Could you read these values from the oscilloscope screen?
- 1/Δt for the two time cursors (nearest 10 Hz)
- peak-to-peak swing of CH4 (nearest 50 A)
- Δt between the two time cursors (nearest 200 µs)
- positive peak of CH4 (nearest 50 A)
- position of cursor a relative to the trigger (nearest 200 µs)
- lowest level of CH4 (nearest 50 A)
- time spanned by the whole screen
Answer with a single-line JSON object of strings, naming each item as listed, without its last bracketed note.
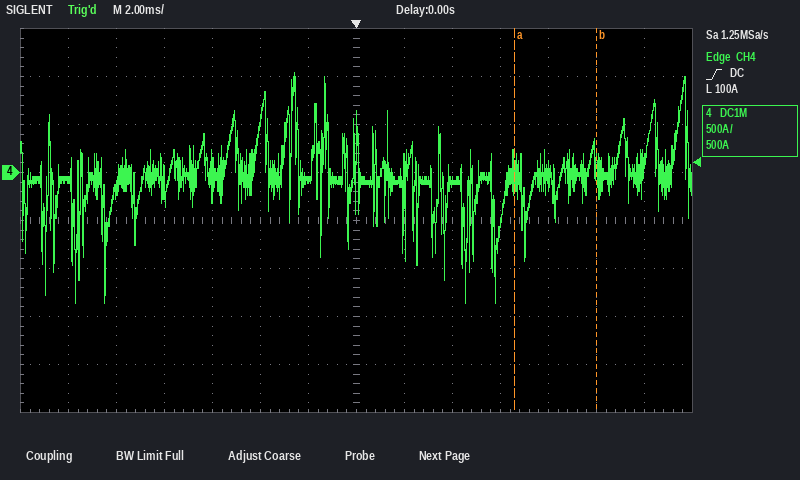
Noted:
{"1/Δt for the two time cursors": "290 Hz", "peak-to-peak swing of CH4": "2.40 kA", "Δt between the two time cursors": "3.4 ms", "positive peak of CH4": "1.05 kA", "position of cursor a relative to the trigger": "+6.6 ms", "lowest level of CH4": "-1.35 kA", "time spanned by the whole screen": "28 ms"}
